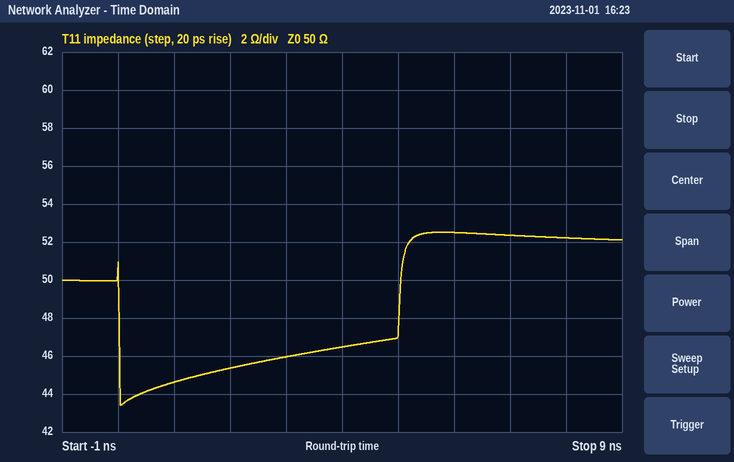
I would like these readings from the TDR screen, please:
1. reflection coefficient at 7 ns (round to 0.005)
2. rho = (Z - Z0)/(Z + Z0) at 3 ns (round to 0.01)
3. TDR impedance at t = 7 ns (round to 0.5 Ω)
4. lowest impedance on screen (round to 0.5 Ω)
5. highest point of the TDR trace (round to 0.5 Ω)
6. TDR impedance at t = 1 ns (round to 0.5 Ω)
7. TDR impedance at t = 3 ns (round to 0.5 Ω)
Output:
+0.025
-0.04
52.5 Ω
43.5 Ω
52.5 Ω
44.5 Ω
46.0 Ω
